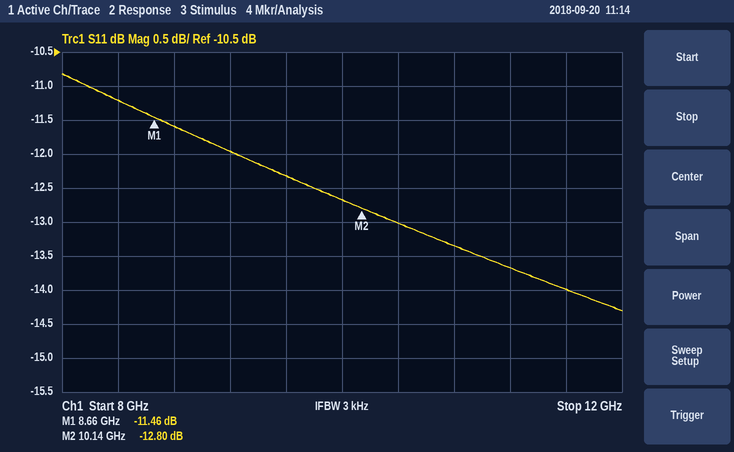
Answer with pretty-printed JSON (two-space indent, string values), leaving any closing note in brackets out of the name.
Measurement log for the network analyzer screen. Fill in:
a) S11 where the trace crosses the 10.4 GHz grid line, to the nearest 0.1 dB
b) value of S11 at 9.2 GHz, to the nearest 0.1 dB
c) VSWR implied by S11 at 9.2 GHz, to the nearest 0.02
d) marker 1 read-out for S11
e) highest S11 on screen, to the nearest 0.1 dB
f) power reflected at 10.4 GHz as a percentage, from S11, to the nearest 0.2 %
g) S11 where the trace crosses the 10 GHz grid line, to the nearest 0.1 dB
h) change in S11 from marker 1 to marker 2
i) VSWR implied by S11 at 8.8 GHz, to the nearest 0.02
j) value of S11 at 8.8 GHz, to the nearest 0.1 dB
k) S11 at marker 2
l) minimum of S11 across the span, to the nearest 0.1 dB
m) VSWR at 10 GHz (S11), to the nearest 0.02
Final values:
{
  "S11 where the trace crosses the 10.4 GHz grid line, to the nearest 0.1 dB": "-13.0 dB",
  "value of S11 at 9.2 GHz, to the nearest 0.1 dB": "-12.0 dB",
  "VSWR implied by S11 at 9.2 GHz, to the nearest 0.02": "1.68",
  "marker 1 read-out for S11": "-11.46 dB",
  "highest S11 on screen, to the nearest 0.1 dB": "-10.8 dB",
  "power reflected at 10.4 GHz as a percentage, from S11, to the nearest 0.2 %": "5.0 %",
  "S11 where the trace crosses the 10 GHz grid line, to the nearest 0.1 dB": "-12.7 dB",
  "change in S11 from marker 1 to marker 2": "-1.34 dB",
  "VSWR implied by S11 at 8.8 GHz, to the nearest 0.02": "1.72",
  "value of S11 at 8.8 GHz, to the nearest 0.1 dB": "-11.6 dB",
  "S11 at marker 2": "-12.80 dB",
  "minimum of S11 across the span, to the nearest 0.1 dB": "-14.3 dB",
  "VSWR at 10 GHz (S11), to the nearest 0.02": "1.60"
}
